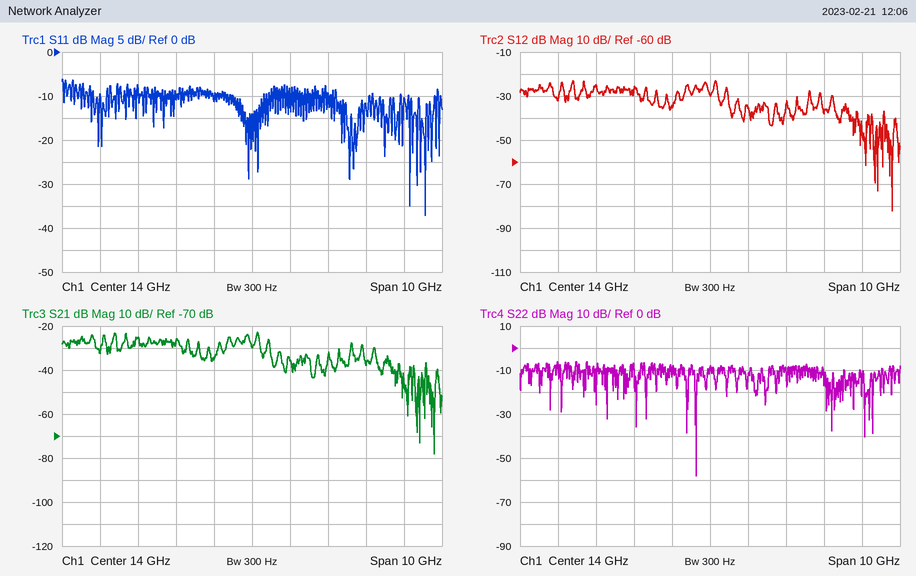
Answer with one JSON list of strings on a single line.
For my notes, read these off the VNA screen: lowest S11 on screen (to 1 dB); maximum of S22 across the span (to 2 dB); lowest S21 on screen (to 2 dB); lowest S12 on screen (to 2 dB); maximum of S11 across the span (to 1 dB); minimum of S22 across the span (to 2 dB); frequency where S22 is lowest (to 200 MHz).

["-37 dB", "-6 dB", "-78 dB", "-82 dB", "-6 dB", "-58 dB", "13.6 GHz"]
